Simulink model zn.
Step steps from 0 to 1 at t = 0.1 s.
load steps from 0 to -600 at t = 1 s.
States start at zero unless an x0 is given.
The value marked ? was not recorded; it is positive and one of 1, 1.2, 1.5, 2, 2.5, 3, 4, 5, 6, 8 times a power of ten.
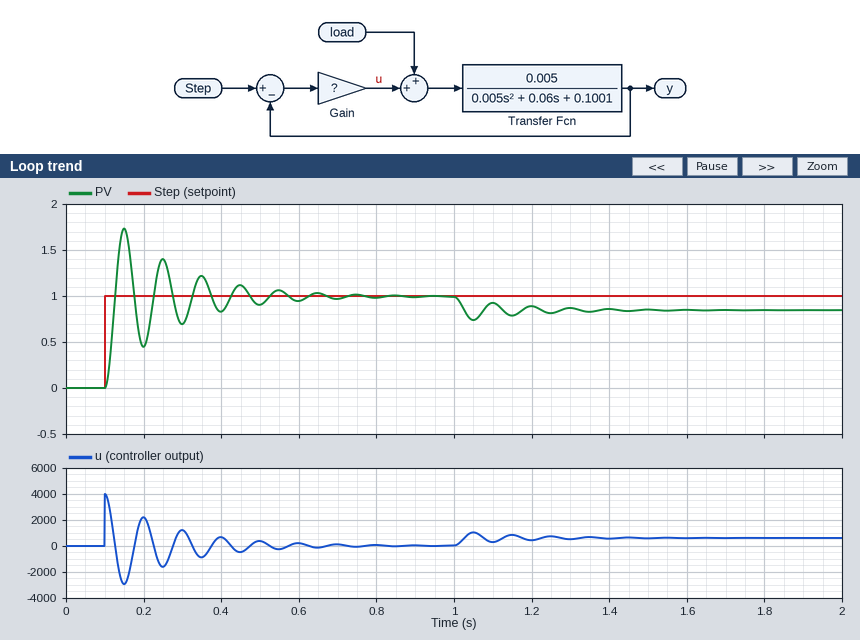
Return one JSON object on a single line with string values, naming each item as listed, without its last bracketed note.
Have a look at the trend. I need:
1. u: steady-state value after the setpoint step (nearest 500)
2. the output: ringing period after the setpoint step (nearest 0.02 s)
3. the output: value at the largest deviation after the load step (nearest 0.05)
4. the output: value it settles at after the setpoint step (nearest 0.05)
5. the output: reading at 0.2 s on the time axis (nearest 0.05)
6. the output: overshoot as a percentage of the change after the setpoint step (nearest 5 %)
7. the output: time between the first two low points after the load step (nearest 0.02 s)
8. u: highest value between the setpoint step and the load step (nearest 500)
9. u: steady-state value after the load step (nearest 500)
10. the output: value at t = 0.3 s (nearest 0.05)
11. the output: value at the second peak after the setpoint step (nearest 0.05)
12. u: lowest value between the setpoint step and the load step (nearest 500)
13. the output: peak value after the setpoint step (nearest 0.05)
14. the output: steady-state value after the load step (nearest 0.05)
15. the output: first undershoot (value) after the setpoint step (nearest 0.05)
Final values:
{"u: steady-state value after the setpoint step": "0", "the output: ringing period after the setpoint step": "0.10 s", "the output: value at the largest deviation after the load step": "0.75", "the output: value it settles at after the setpoint step": "1.00", "the output: reading at 0.2 s on the time axis": "0.45", "the output: overshoot as a percentage of the change after the setpoint step": "75 %", "the output: time between the first two low points after the load step": "0.10 s", "u: highest value between the setpoint step and the load step": "4000", "u: steady-state value after the load step": "500", "the output: value at t = 0.3 s": "0.70", "the output: value at the second peak after the setpoint step": "1.40", "u: lowest value between the setpoint step and the load step": "-3000", "the output: peak value after the setpoint step": "1.75", "the output: steady-state value after the load step": "0.85", "the output: first undershoot (value) after the setpoint step": "0.45"}
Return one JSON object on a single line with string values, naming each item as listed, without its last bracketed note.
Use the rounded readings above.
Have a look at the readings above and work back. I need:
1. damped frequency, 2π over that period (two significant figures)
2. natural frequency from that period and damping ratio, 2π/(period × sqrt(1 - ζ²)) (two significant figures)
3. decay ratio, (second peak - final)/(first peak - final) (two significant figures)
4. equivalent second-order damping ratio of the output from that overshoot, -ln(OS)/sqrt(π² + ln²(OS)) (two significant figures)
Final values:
{"damped frequency, 2π over that period": "63 rad/s", "natural frequency from that period and damping ratio, 2π/(period × sqrt(1 - ζ²))": "63 rad/s", "decay ratio, (second peak - final)/(first peak - final)": "0.53", "equivalent second-order damping ratio of the output from that overshoot, -ln(OS)/sqrt(π² + ln²(OS))": "0.091"}
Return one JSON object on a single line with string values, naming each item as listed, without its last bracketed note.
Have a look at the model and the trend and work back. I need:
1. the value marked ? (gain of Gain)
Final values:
{"the value marked ?": "4000"}
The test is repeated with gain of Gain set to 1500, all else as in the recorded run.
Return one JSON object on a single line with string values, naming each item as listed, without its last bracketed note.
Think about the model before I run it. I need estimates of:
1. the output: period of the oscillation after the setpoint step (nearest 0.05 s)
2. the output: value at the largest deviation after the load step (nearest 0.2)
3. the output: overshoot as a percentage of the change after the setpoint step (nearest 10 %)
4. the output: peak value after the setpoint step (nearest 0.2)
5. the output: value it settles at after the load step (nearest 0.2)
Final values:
{"the output: period of the oscillation after the setpoint step": "0.15 s", "the output: value at the largest deviation after the load step": "0.4", "the output: overshoot as a percentage of the change after the setpoint step": "60 %", "the output: peak value after the setpoint step": "1.6", "the output: value it settles at after the load step": "0.6"}
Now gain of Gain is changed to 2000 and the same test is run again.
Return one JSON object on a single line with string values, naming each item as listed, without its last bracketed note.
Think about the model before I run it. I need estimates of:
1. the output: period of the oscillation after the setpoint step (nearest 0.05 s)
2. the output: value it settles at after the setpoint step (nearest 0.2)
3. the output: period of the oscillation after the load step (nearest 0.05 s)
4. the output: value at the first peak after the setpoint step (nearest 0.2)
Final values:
{"the output: period of the oscillation after the setpoint step": "0.15 s", "the output: value it settles at after the setpoint step": "1.0", "the output: period of the oscillation after the load step": "0.15 s", "the output: value at the first peak after the setpoint step": "1.6"}
